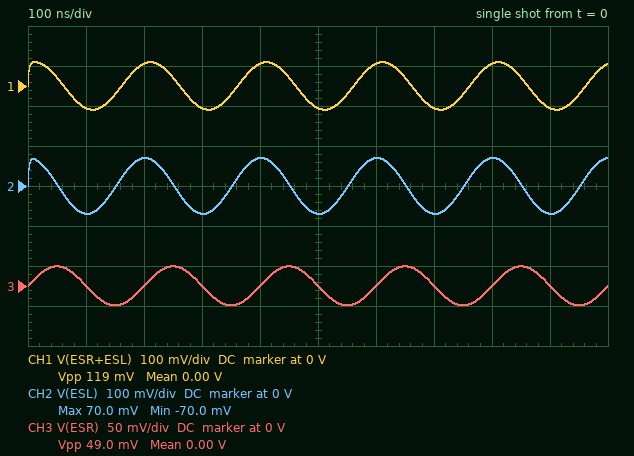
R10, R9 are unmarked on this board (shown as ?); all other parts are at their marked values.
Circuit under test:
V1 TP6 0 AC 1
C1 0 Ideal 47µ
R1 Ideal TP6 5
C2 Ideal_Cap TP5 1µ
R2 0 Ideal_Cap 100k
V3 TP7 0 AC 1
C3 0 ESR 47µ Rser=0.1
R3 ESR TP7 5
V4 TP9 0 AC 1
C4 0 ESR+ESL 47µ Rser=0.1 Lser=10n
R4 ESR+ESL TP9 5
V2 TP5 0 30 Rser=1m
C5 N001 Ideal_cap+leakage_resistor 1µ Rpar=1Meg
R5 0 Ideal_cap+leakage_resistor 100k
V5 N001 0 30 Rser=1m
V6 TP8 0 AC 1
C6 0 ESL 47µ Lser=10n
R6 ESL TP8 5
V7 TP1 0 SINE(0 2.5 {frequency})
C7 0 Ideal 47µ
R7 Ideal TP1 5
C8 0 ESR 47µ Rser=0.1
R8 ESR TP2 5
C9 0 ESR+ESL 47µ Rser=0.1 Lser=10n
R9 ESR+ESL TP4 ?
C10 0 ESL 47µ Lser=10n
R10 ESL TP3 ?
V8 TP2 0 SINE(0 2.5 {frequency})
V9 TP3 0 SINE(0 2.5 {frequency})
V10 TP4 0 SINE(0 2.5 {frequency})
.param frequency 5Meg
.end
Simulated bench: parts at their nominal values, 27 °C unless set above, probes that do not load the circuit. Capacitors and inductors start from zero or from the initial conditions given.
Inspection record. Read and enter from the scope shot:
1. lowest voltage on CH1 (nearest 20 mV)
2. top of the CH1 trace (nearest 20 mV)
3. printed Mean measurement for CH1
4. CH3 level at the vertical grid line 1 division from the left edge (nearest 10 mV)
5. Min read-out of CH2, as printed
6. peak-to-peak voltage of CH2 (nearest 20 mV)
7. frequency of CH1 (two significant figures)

-60 mV
60 mV
0.00 V
0 V
-70.0 mV
140 mV
5.0 MHz
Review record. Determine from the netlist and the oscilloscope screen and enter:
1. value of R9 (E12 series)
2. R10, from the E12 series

6.8 Ω
5.6 Ω
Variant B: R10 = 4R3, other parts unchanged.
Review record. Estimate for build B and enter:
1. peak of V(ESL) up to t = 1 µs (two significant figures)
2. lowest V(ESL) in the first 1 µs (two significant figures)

91 mV
-91 mV
